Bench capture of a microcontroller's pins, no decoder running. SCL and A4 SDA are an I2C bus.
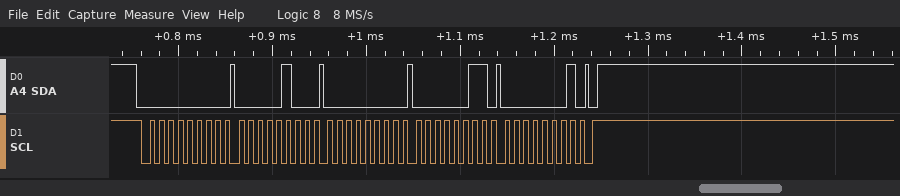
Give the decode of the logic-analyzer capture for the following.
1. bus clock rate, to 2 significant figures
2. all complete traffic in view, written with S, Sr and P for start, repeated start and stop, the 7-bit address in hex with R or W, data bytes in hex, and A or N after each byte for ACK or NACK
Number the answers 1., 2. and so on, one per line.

1. 100 kHz
2. S 00W A 04 A 00 A 03 A 01 A P
